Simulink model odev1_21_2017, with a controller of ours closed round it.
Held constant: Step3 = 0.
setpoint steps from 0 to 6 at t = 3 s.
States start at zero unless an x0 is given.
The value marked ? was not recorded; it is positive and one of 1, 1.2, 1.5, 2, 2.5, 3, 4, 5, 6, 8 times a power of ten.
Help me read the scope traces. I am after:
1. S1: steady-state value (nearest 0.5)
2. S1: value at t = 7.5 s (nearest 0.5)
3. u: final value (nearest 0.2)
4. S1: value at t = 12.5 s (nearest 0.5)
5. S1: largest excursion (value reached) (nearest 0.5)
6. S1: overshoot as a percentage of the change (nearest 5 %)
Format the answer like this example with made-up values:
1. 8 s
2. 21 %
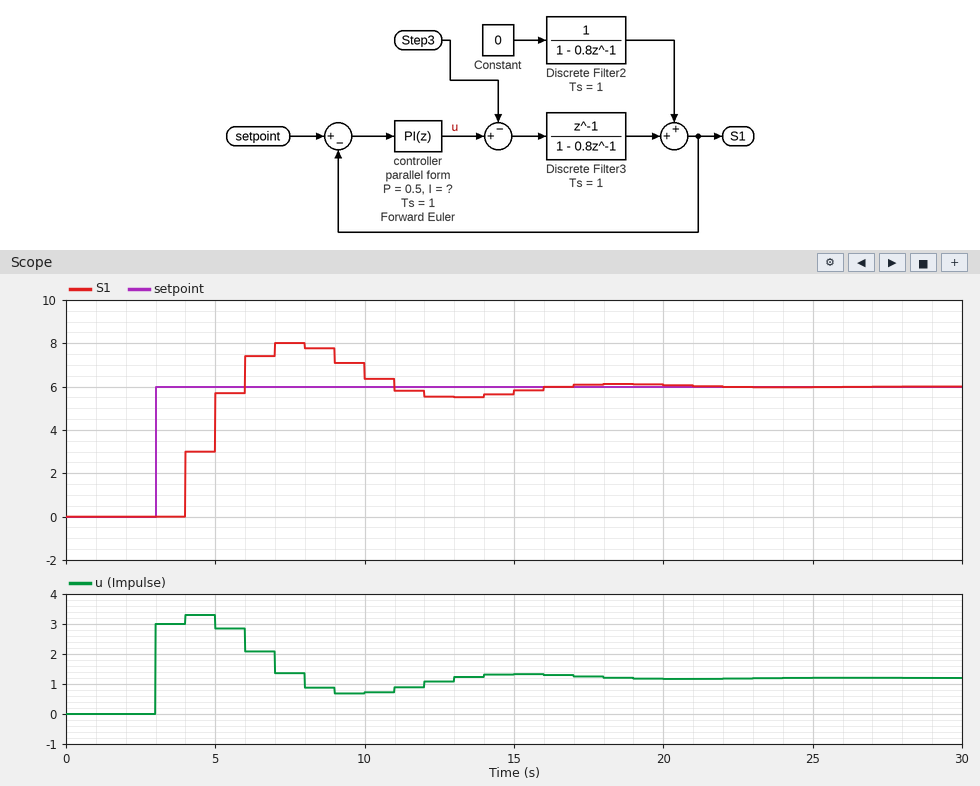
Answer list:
1. 6.0
2. 8.0
3. 1.2
4. 5.5
5. 8.0
6. 35 %
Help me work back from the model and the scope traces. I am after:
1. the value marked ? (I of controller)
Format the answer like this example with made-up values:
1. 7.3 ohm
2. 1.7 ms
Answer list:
1. 0.3
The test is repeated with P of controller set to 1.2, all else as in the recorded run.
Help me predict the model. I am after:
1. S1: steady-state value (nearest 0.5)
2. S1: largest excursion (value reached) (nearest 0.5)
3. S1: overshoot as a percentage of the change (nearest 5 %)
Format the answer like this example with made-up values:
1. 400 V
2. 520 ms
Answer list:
1. 6.0
2. 7.0
3. 20 %
